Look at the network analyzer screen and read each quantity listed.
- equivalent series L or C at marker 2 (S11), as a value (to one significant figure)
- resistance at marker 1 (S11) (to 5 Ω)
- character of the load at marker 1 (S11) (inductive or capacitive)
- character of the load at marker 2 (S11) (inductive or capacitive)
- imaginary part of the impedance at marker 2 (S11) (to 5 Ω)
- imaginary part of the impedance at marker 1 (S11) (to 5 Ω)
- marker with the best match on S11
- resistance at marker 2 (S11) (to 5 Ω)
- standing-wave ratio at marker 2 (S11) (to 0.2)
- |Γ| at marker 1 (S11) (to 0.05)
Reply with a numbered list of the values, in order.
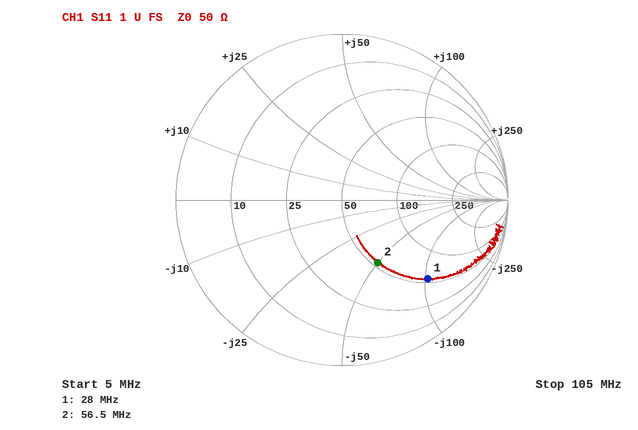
1. 60 pF
2. 55 Ω
3. capacitive
4. capacitive
5. -50 Ω
6. -105 Ω
7. marker 2
8. 55 Ω
9. 2.6
10. 0.70
